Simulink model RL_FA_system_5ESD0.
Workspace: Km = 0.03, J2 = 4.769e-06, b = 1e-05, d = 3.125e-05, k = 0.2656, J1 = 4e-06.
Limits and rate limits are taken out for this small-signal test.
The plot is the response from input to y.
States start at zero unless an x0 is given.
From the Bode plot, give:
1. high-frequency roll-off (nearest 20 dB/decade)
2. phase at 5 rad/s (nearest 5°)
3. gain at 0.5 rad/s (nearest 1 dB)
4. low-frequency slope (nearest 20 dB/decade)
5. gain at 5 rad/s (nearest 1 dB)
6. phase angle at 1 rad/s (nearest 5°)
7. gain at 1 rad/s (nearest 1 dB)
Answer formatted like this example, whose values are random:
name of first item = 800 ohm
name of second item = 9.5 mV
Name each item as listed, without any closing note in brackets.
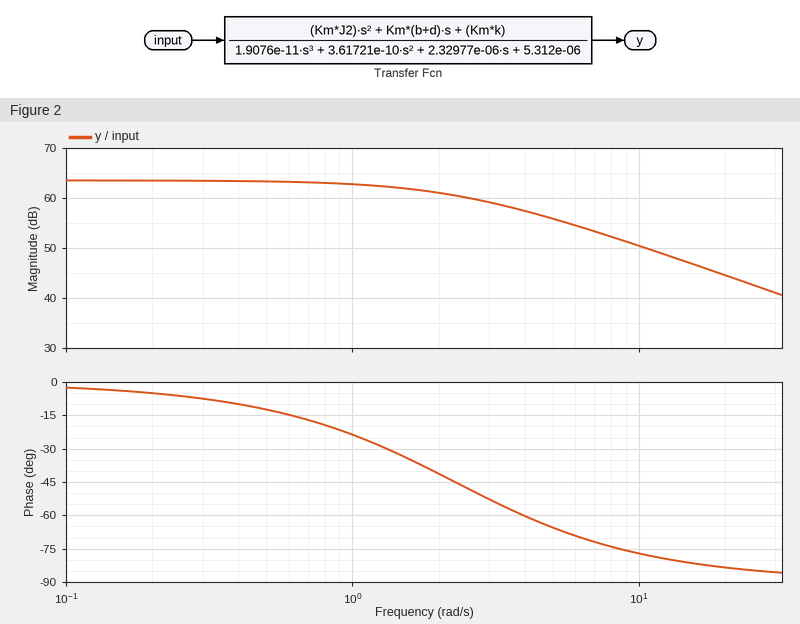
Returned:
high-frequency roll-off = -20 dB/decade
phase at 5 rad/s = -65°
gain at 0.5 rad/s = 63 dB
low-frequency slope = 0 dB/decade
gain at 5 rad/s = 56 dB
phase angle at 1 rad/s = -25°
gain at 1 rad/s = 63 dB
